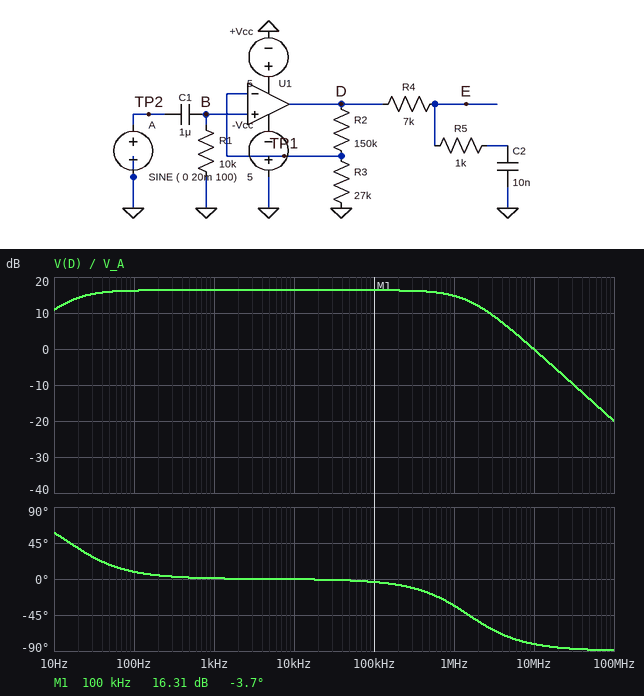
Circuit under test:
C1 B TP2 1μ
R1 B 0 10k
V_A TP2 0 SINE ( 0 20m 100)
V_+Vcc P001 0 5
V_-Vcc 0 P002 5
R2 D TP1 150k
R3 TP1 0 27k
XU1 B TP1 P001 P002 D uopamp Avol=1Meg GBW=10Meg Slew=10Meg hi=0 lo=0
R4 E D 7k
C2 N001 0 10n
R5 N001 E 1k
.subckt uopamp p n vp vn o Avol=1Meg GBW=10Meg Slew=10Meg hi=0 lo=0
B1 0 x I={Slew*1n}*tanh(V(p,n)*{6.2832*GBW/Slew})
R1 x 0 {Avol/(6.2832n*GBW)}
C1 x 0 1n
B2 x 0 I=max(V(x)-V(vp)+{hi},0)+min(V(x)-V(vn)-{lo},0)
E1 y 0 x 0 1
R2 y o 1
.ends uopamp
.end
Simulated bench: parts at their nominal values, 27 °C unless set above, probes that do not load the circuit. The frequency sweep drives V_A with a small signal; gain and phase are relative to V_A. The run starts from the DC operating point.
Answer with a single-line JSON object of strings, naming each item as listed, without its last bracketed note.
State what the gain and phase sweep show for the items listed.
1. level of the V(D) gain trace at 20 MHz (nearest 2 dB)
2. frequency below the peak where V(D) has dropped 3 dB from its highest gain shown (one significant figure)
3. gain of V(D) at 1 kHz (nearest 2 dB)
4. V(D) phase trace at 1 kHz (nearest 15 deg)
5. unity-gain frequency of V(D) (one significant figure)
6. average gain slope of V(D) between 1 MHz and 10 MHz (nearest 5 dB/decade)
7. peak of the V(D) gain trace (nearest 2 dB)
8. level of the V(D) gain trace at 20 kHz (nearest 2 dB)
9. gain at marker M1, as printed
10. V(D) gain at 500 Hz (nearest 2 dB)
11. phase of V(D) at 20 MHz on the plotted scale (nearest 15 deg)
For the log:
{"level of the V(D) gain trace at 20 MHz": "-6 dB", "frequency below the peak where V(D) has dropped 3 dB from its highest gain shown": "20 Hz", "gain of V(D) at 1 kHz": "16 dB", "V(D) phase trace at 1 kHz": "0 deg", "unity-gain frequency of V(D)": "10 MHz", "average gain slope of V(D) between 1 MHz and 10 MHz": "-15 dB/decade", "peak of the V(D) gain trace": "16 dB", "level of the V(D) gain trace at 20 kHz": "16 dB", "gain at marker M1, as printed": "16.31 dB", "V(D) gain at 500 Hz": "16 dB", "phase of V(D) at 20 MHz on the plotted scale": "-90 deg"}
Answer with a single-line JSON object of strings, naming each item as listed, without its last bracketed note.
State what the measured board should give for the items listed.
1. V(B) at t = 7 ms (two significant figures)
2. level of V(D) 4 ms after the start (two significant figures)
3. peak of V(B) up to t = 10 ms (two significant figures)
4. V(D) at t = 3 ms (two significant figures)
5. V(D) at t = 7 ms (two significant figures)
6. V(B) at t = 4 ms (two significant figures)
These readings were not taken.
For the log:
{"V(B) at t = 7 ms": "-21 mV", "level of V(D) 4 ms after the start": "45 mV", "peak of V(B) up to t = 10 ms": "17 mV", "V(D) at t = 3 ms": "100 mV", "V(D) at t = 7 ms": "-140 mV", "V(B) at t = 4 ms": "6.9 mV"}
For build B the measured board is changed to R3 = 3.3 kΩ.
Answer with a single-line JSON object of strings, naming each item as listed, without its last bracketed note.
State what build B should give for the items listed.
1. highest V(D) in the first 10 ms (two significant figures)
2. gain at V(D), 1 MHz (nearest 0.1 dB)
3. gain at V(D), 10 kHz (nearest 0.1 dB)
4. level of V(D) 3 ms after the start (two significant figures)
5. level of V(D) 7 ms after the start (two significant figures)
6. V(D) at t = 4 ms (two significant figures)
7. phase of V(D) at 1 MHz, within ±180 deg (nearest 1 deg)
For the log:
{"highest V(D) in the first 10 ms": "800 mV", "gain at V(D), 1 MHz": "19.8 dB", "gain at V(D), 10 kHz": "33.3 dB", "level of V(D) 3 ms after the start": "710 mV", "level of V(D) 7 ms after the start": "-980 mV", "V(D) at t = 4 ms": "320 mV", "phase of V(D) at 1 MHz, within ±180 deg": "-78 deg"}
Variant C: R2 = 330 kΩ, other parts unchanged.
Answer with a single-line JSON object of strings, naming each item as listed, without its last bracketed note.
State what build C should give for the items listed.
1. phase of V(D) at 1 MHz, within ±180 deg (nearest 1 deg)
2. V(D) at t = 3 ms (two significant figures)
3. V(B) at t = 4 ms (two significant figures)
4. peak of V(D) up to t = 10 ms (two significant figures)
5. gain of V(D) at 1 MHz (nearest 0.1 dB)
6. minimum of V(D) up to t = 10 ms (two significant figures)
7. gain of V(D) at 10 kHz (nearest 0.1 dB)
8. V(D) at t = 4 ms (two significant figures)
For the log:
{"phase of V(D) at 1 MHz, within ±180 deg": "-53 deg", "V(D) at t = 3 ms": "200 mV", "V(B) at t = 4 ms": "6.9 mV", "peak of V(D) up to t = 10 ms": "230 mV", "gain of V(D) at 1 MHz": "18.0 dB", "minimum of V(D) up to t = 10 ms": "-280 mV", "gain of V(D) at 10 kHz": "22.4 dB", "V(D) at t = 4 ms": "91 mV"}
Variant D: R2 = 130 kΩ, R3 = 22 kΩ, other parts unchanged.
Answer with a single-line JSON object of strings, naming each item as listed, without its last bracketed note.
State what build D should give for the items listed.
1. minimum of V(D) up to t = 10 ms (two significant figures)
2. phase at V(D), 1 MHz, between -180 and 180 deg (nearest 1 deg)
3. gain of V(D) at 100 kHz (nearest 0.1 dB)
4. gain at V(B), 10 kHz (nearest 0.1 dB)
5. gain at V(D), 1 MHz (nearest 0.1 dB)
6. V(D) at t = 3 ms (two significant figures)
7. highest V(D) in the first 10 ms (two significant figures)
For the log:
{"minimum of V(D) up to t = 10 ms": "-150 mV", "phase at V(D), 1 MHz, between -180 and 180 deg": "-35 deg", "gain of V(D) at 100 kHz": "16.8 dB", "gain at V(B), 10 kHz": "0 dB", "gain at V(D), 1 MHz": "15.1 dB", "V(D) at t = 3 ms": "110 mV", "highest V(D) in the first 10 ms": "120 mV"}
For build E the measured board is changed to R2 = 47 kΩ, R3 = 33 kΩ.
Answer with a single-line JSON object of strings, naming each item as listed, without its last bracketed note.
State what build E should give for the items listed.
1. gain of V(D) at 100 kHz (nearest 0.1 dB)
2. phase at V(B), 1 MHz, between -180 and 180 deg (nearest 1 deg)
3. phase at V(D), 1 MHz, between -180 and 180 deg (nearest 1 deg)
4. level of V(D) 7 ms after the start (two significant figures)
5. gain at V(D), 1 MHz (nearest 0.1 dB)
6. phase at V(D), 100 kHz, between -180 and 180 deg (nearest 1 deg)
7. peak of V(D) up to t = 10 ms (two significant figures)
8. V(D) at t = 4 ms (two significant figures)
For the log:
{"gain of V(D) at 100 kHz": "7.7 dB", "phase at V(B), 1 MHz, between -180 and 180 deg": "0 deg", "phase at V(D), 1 MHz, between -180 and 180 deg": "-14 deg", "level of V(D) 7 ms after the start": "-51 mV", "gain at V(D), 1 MHz": "7.4 dB", "phase at V(D), 100 kHz, between -180 and 180 deg": "-1 deg", "peak of V(D) up to t = 10 ms": "42 mV", "V(D) at t = 4 ms": "17 mV"}
